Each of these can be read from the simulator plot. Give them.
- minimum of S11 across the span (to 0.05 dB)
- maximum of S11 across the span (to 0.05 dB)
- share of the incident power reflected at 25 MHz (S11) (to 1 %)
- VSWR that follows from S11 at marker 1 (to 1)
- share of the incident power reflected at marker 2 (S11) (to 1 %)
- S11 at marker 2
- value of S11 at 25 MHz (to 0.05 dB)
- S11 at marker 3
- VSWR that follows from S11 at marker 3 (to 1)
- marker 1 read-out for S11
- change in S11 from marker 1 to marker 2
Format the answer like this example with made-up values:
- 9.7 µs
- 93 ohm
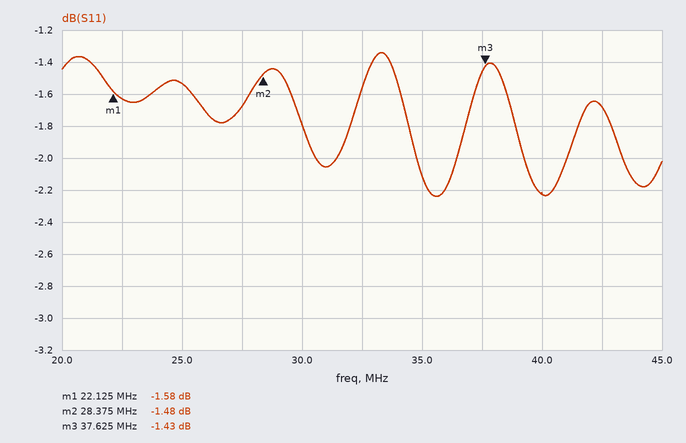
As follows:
- -2.25 dB
- -1.35 dB
- 70 %
- 11
- 71 %
- -1.48 dB
- -1.55 dB
- -1.43 dB
- 12
- -1.58 dB
- 0.10 dB
